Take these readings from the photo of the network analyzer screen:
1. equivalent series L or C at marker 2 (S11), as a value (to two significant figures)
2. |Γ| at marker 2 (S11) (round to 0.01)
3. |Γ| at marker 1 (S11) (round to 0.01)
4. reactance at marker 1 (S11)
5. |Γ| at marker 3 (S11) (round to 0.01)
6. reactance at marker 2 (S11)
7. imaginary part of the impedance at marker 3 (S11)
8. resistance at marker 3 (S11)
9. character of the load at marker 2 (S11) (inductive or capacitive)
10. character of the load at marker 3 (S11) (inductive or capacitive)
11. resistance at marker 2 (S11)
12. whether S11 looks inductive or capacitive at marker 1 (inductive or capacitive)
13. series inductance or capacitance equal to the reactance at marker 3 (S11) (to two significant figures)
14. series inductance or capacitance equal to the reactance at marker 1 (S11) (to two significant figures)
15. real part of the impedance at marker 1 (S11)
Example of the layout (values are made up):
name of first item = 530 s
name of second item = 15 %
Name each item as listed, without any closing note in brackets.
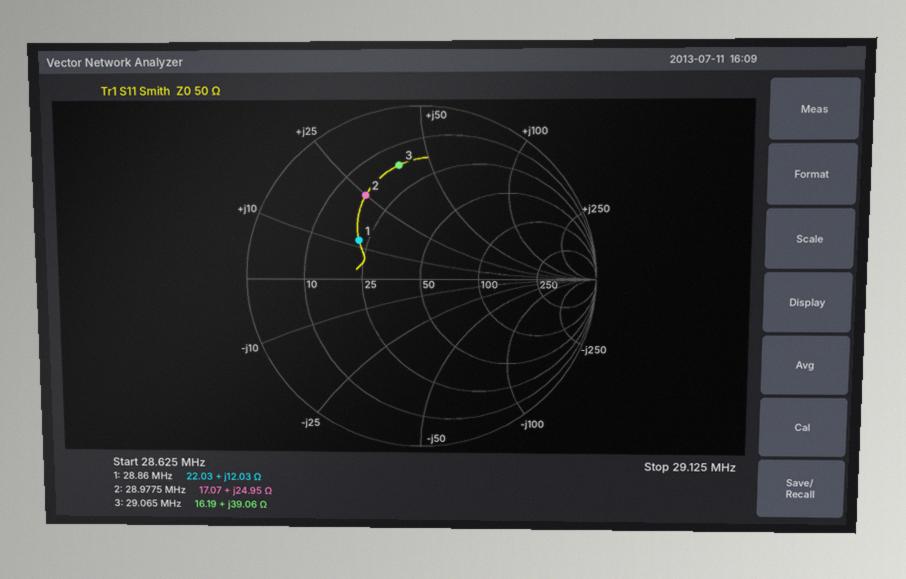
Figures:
equivalent series L or C at marker 2 (S11), as a value = 140 nH
|Γ| at marker 2 (S11) = 0.58
|Γ| at marker 1 (S11) = 0.42
reactance at marker 1 = +12.03 Ω
|Γ| at marker 3 (S11) = 0.67
reactance at marker 2 = +24.95 Ω
imaginary part of the impedance at marker 3 = +39.06 Ω
resistance at marker 3 = 16.19 Ω
character of the load at marker 2 (S11) = inductive
character of the load at marker 3 (S11) = inductive
resistance at marker 2 = 17.07 Ω
whether S11 looks inductive or capacitive at marker 1 = inductive
series inductance or capacitance equal to the reactance at marker 3 (S11) = 210 nH
series inductance or capacitance equal to the reactance at marker 1 (S11) = 66 nH
real part of the impedance at marker 1 = 22.03 Ω
